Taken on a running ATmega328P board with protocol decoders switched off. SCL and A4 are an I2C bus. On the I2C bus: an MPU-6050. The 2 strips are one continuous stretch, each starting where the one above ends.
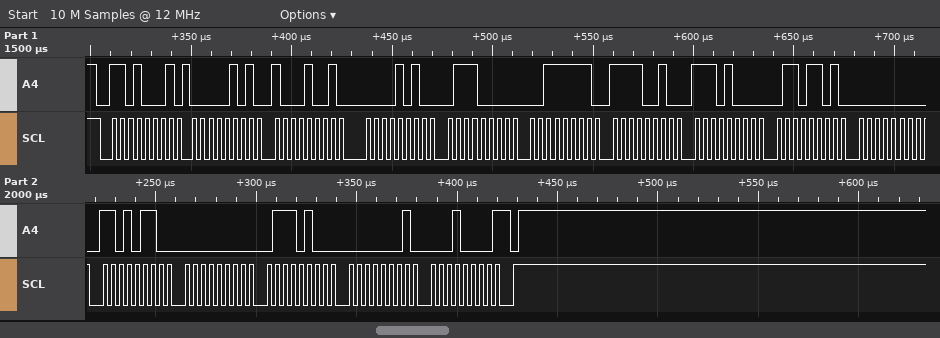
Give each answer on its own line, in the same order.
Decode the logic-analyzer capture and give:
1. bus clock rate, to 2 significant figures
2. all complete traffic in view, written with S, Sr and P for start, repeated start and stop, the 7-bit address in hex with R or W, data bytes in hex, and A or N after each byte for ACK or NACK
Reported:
250 kHz
S 68R A 05 A 89 A 0A A 70 A 3F A F2 A E8 A 6D A 00 A D6 A 00 A 74 A 01 A 10 N P
